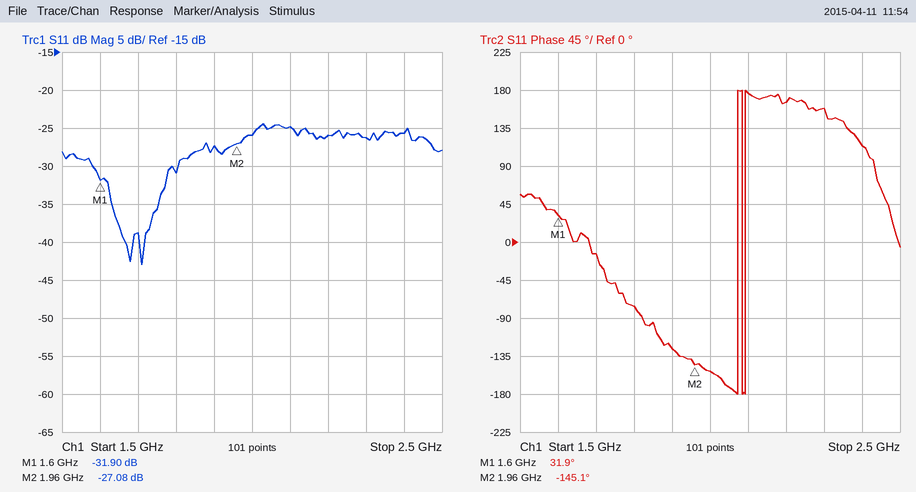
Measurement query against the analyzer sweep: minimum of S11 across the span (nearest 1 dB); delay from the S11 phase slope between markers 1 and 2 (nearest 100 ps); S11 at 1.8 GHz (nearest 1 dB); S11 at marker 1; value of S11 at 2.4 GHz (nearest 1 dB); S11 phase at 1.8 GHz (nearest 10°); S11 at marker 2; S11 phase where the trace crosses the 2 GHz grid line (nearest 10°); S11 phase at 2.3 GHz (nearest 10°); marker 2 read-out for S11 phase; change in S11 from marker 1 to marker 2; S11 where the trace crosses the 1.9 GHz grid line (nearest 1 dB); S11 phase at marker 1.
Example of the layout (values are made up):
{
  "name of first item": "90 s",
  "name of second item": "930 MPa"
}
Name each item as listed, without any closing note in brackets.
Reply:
{
  "minimum of S11 across the span": "-43 dB",
  "delay from the S11 phase slope between markers 1 and 2": "1.4 ns",
  "S11 at 1.8 GHz": "-31 dB",
  "S11 at marker 1": "-31.90 dB",
  "value of S11 at 2.4 GHz": "-26 dB",
  "S11 phase at 1.8 GHz": "-80°",
  "S11 at marker 2": "-27.08 dB",
  "S11 phase where the trace crosses the 2 GHz grid line": "-150°",
  "S11 phase at 2.3 GHz": "160°",
  "marker 2 read-out for S11 phase": "-145.1°",
  "change in S11 from marker 1 to marker 2": "4.82 dB",
  "S11 where the trace crosses the 1.9 GHz grid line": "-27 dB",
  "S11 phase at marker 1": "31.9°"
}
